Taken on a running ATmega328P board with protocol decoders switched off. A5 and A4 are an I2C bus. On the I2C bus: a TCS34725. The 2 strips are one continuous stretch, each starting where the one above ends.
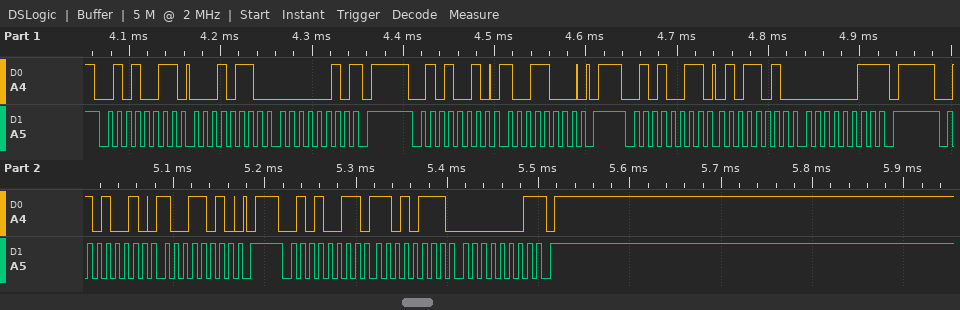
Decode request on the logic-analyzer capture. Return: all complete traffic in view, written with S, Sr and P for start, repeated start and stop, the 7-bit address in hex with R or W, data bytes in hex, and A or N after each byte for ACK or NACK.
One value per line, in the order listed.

S 29R A 16 A 02 N P S 29W A 98 A P S 29R A 5A A 03 N P S 29W A 9A A P S 29R A D7 A 01 N P
